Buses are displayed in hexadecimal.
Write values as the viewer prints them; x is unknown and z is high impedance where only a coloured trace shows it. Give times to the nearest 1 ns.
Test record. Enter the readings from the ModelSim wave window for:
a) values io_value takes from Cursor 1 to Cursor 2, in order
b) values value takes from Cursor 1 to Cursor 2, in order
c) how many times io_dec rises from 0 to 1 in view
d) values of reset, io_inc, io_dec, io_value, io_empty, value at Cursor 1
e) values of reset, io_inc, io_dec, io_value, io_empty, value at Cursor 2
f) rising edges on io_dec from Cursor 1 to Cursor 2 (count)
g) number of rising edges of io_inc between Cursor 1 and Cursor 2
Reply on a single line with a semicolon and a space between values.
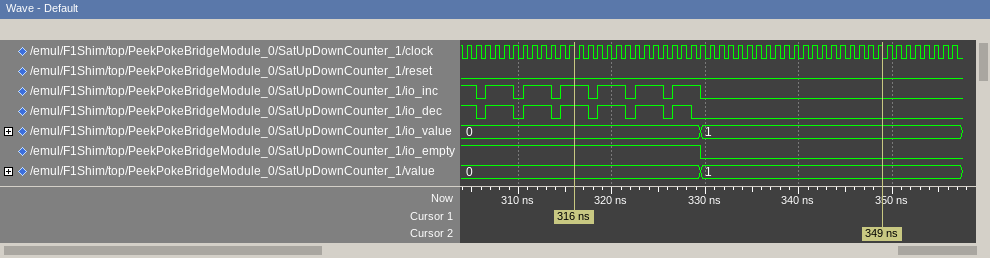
0, 1; 0, 1; 6; reset=0, io_inc=1, io_dec=1, io_value=0, io_empty=1, value=0; reset=0, io_inc=0, io_dec=0, io_value=1, io_empty=0, value=1; 3; 3
